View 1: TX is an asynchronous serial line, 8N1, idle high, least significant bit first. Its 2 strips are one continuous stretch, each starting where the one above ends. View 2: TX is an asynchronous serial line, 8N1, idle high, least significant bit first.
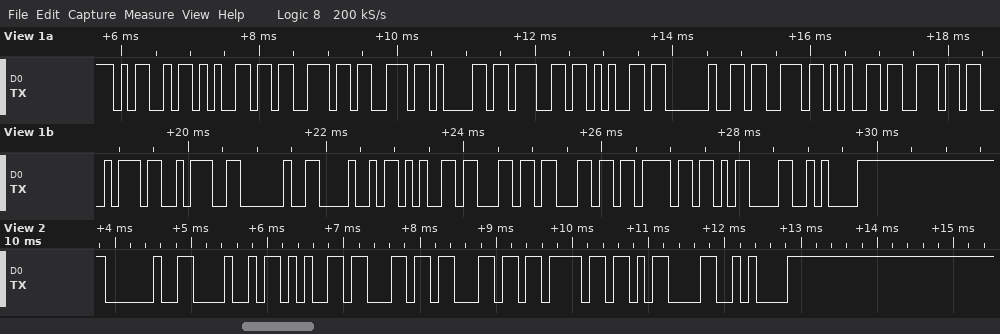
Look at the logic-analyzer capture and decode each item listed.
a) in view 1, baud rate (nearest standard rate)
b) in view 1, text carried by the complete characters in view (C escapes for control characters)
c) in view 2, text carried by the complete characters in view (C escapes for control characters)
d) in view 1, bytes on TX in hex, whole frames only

9600 baud
"Message sent: Hello\r\n"
" Hello\r\n"
4D 65 73 73 61 67 65 20 73 65 6E 74 3A 20 48 65 6C 6C 6F 0D 0A
